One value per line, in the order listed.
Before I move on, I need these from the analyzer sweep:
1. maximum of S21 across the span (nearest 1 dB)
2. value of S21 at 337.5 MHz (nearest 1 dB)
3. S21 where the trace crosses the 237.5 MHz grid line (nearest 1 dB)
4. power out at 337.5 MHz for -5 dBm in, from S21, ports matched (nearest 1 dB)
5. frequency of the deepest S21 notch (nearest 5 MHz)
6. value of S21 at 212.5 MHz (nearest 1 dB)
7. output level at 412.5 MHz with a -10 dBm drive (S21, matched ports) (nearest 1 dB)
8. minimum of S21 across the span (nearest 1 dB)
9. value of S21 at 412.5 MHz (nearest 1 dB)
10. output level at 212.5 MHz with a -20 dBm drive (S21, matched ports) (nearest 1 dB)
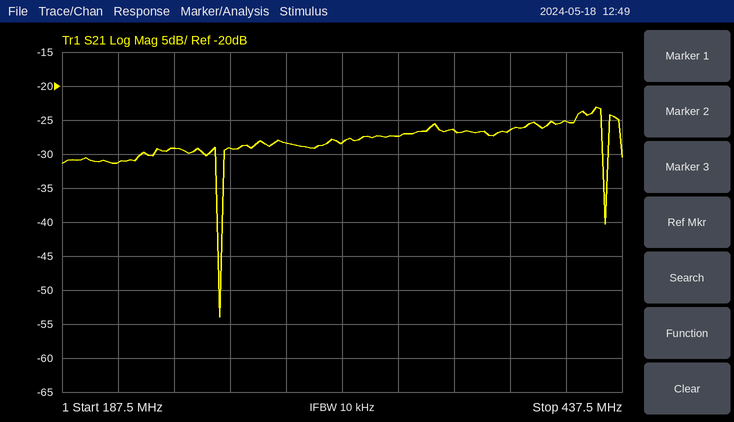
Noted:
-23 dB
-27 dB
-29 dB
-32 dBm
260 MHz
-31 dB
-35 dBm
-54 dB
-25 dB
-51 dBm
